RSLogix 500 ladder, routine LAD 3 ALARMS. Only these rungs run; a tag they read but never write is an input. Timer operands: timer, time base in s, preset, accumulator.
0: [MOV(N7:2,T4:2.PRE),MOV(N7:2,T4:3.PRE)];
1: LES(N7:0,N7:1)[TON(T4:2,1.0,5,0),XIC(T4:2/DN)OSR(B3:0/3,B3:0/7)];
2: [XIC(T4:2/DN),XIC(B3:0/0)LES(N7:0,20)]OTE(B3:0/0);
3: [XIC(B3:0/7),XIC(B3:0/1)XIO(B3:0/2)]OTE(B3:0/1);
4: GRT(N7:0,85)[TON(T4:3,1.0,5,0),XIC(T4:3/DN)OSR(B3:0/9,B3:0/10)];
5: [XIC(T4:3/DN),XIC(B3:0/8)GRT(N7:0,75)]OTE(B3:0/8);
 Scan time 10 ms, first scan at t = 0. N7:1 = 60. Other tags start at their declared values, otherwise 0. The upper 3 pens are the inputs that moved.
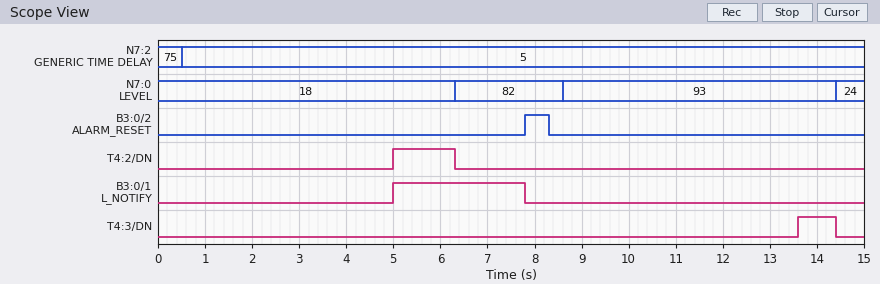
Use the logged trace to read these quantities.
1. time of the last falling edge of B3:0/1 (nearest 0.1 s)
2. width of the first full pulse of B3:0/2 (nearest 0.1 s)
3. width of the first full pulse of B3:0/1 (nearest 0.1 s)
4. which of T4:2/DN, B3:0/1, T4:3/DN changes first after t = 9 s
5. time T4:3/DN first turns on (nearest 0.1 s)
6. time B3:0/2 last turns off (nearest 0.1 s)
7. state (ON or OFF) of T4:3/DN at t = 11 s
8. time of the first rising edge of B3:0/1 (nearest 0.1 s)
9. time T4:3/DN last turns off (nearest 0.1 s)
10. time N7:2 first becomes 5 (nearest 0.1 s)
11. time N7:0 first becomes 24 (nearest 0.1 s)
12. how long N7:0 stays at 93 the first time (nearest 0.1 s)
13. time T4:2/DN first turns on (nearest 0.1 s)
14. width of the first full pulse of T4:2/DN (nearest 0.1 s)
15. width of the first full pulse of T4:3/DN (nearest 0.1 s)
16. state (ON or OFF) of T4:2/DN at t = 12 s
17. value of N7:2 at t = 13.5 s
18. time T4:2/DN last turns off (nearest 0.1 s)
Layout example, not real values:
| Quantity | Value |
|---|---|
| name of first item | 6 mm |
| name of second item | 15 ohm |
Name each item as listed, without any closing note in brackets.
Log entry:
| Quantity | Value |
|---|---|
| time of the last falling edge of B3:0/1 | 7.8 s |
| width of the first full pulse of B3:0/2 | 0.5 s |
| width of the first full pulse of B3:0/1 | 2.8 s |
| which of T4:2/DN, B3:0/1, T4:3/DN changes first after t = 9 s | T4:3/DN |
| time T4:3/DN first turns on | 13.6 s |
| time B3:0/2 last turns off | 8.3 s |
| state (ON or OFF) of T4:3/DN at t = 11 s | OFF |
| time of the first rising edge of B3:0/1 | 5.0 s |
| time T4:3/DN last turns off | 14.4 s |
| time N7:2 first becomes 5 | 0.5 s |
| time N7:0 first becomes 24 | 14.4 s |
| how long N7:0 stays at 93 the first time | 5.8 s |
| time T4:2/DN first turns on | 5.0 s |
| width of the first full pulse of T4:2/DN | 1.3 s |
| width of the first full pulse of T4:3/DN | 0.8 s |
| state (ON or OFF) of T4:2/DN at t = 12 s | OFF |
| value of N7:2 at t = 13.5 s | 5 |
| time T4:2/DN last turns off | 6.3 s |
